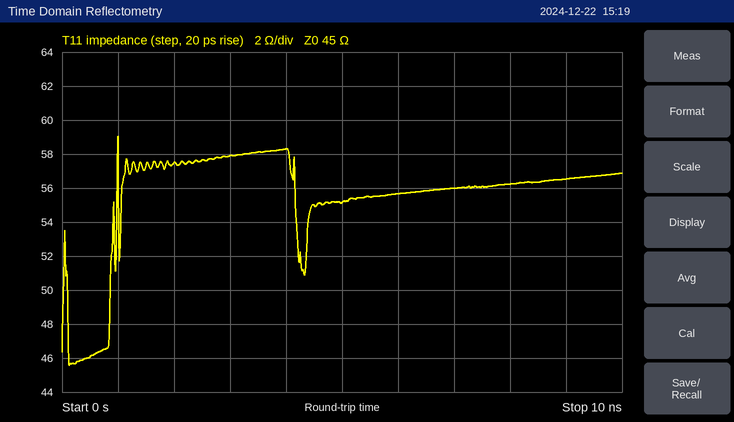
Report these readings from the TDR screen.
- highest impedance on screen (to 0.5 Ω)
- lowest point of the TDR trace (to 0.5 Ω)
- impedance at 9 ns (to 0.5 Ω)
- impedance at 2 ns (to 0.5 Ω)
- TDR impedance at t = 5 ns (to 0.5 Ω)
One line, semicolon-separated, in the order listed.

59.0 Ω; 45.5 Ω; 56.5 Ω; 57.5 Ω; 55.0 Ω
